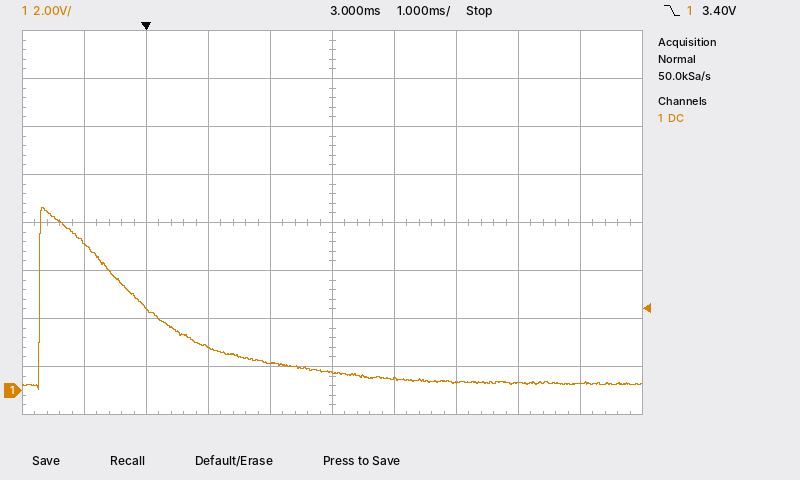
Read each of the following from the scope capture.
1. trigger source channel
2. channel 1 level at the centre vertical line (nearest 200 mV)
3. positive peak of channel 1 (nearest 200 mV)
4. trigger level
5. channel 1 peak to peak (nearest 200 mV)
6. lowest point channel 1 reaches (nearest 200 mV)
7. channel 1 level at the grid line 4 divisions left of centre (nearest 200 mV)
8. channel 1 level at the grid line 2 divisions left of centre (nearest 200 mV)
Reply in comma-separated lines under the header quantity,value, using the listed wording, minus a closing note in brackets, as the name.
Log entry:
quantity,value
trigger source channel,channel 1
channel 1 level at the centre vertical line,800 mV
positive peak of channel 1,7.6 V
trigger level,3.40 V
channel 1 peak to peak,7.6 V
lowest point channel 1 reaches,0.0 V
channel 1 level at the grid line 4 divisions left of centre,6.2 V
channel 1 level at the grid line 2 divisions left of centre,1.8 V
